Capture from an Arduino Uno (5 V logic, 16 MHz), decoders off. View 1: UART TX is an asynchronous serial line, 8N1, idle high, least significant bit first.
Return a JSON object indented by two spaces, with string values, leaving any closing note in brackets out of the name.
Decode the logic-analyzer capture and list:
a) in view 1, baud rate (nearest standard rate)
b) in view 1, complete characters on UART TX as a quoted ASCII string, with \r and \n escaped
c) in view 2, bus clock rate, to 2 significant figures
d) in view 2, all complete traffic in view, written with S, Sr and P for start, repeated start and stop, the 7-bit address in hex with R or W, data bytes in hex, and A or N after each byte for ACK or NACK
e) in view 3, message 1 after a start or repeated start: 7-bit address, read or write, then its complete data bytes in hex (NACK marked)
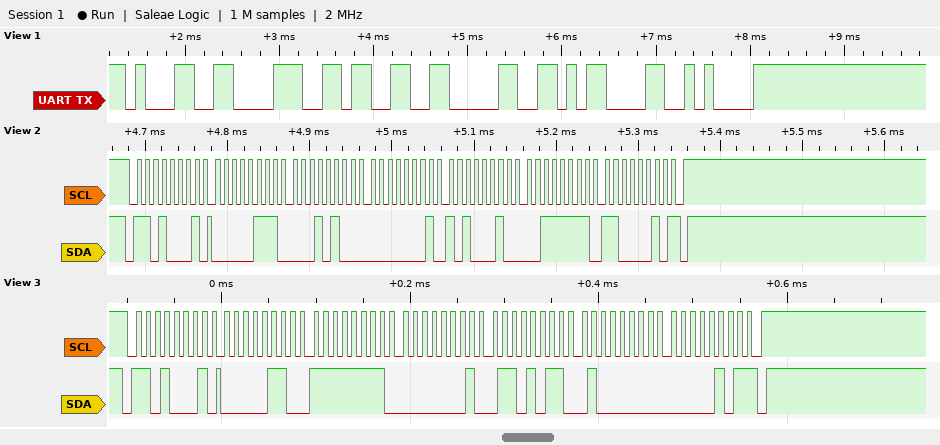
{
  "in view 1, baud rate": "9600 baud",
  "in view 1, complete characters on UART TX as a quoted ASCII string, with \\r and \\n escaped": "\"1830\\r\\n\"",
  "in view 2, bus clock rate, to 2 significant figures": "100 kHz",
  "in view 2, all complete traffic in view, written with S, Sr and P for start, repeated start and stop, the 7-bit address in hex with R or W, data bytes in hex, and A or N after each byte for ACK or NACK": "S 68R A 07 A 14 A 01 A A2 A 3F A C2 N P",
  "in view 3, message 1 after a start or repeated start: 7-bit address, read or write, then its complete data bytes in hex": "0x68 read: 06 FF 01 6B 40 05 NACK"
}
